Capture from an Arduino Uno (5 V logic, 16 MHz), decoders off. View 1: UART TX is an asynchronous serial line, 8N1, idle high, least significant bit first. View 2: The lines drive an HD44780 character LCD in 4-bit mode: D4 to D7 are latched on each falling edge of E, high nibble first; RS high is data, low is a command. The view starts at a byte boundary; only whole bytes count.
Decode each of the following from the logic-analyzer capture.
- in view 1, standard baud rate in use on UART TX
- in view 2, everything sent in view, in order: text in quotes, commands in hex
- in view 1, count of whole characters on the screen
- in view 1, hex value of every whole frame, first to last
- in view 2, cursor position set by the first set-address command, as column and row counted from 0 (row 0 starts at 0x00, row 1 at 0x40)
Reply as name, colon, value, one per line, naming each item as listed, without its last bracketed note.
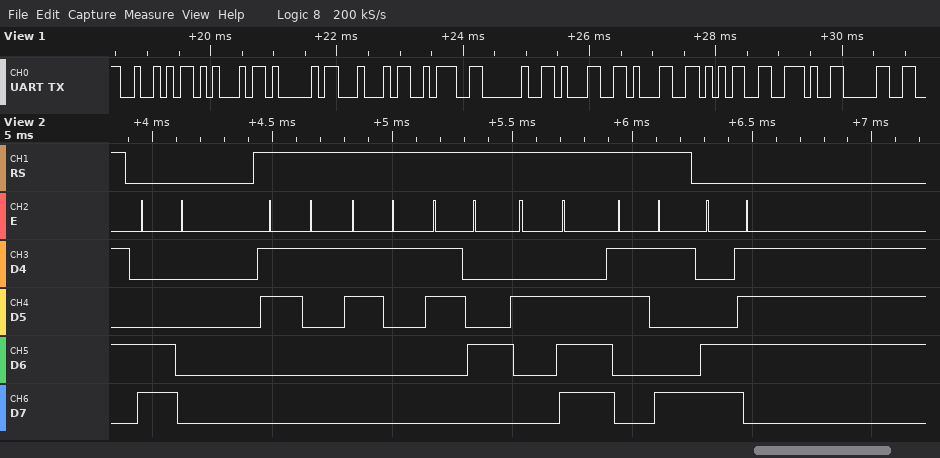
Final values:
in view 1, standard baud rate in use on UART TX: 9600 baud
in view 2, everything sent in view, in order: text in quotes, commands in hex: 0xC0 "114.9" 0xC7
in view 1, count of whole characters on the screen: 11
in view 1, hex value of every whole frame, first to last: 52 45 41 44 3A 20 31 31 35 2E 30
in view 2, cursor position set by the first set-address command, as column and row counted from 0: column 0, row 1
